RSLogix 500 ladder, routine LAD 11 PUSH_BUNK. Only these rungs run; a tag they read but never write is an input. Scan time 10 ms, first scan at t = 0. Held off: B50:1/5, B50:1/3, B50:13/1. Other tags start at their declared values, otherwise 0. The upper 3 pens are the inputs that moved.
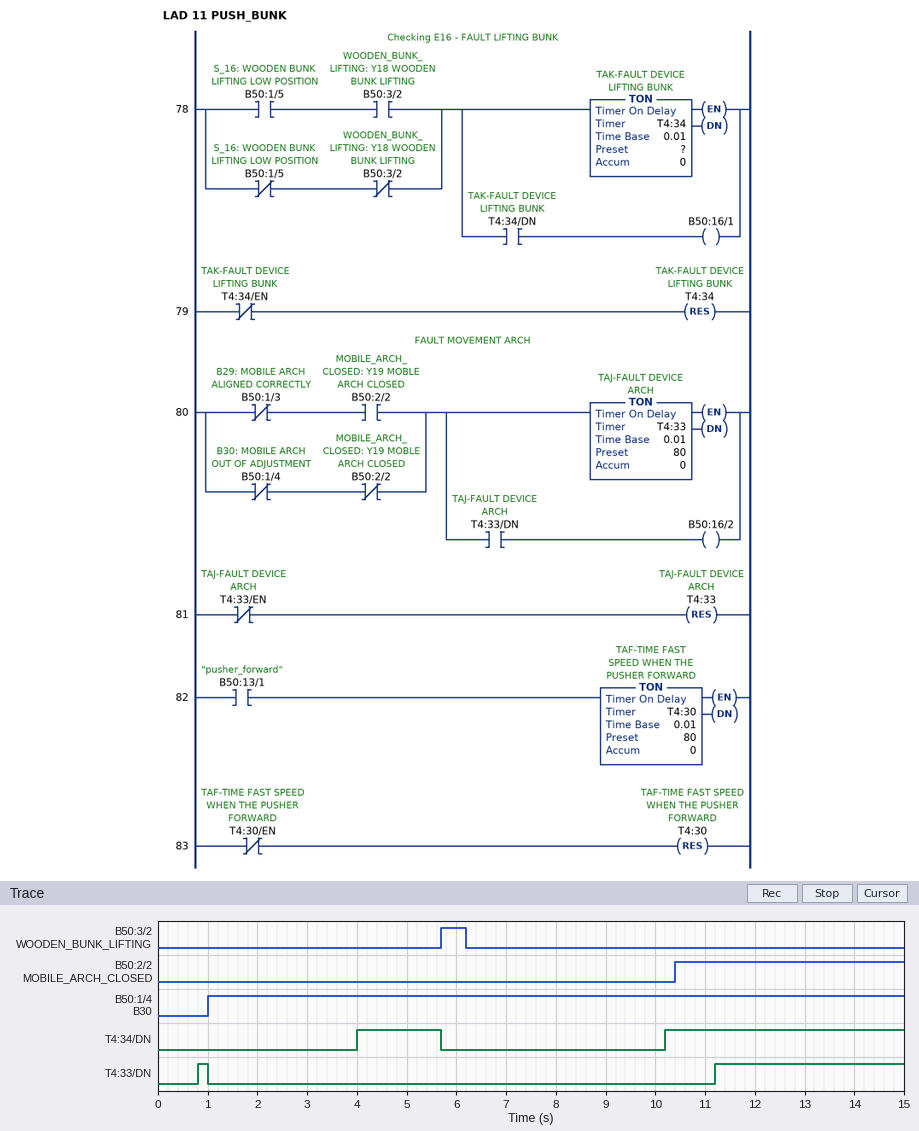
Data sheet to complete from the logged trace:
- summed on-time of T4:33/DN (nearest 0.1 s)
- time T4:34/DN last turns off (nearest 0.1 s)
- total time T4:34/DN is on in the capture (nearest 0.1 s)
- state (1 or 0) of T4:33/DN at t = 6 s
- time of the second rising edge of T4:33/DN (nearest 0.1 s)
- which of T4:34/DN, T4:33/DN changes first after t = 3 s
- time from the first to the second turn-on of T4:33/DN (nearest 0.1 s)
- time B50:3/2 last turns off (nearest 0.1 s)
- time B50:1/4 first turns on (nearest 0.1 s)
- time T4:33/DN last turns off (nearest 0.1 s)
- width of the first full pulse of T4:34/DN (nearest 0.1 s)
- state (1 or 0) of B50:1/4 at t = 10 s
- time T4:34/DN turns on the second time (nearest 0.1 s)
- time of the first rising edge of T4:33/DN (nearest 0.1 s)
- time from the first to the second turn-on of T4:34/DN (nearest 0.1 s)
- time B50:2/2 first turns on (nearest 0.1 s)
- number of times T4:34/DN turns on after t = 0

4.0 s
5.7 s
6.5 s
0
11.2 s
T4:34/DN
10.4 s
6.2 s
1.0 s
1.0 s
1.7 s
1
10.2 s
0.8 s
6.2 s
10.4 s
2
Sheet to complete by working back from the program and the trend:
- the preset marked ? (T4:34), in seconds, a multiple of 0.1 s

4.0 s
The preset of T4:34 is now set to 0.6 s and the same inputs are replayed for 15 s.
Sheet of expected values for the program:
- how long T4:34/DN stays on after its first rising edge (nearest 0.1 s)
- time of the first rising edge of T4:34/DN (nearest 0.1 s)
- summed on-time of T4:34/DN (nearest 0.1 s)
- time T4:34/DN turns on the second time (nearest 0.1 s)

5.1 s
0.6 s
13.3 s
6.8 s
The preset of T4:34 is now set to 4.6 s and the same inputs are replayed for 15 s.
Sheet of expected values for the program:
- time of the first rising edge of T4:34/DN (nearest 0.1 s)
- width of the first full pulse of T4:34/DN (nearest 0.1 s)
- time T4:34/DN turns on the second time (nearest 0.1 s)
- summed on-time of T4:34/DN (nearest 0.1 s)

4.6 s
1.1 s
10.8 s
5.3 s
